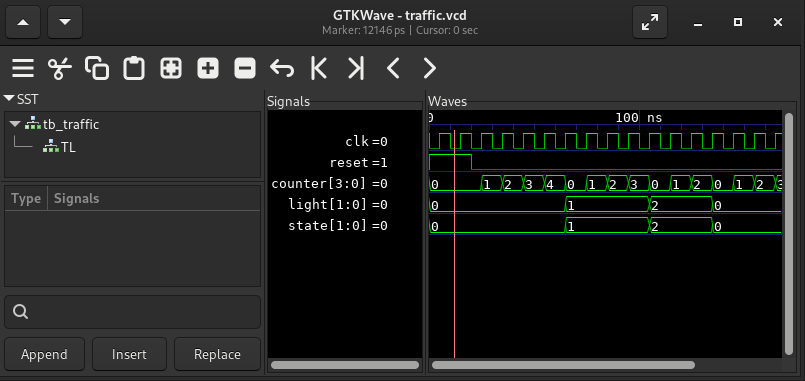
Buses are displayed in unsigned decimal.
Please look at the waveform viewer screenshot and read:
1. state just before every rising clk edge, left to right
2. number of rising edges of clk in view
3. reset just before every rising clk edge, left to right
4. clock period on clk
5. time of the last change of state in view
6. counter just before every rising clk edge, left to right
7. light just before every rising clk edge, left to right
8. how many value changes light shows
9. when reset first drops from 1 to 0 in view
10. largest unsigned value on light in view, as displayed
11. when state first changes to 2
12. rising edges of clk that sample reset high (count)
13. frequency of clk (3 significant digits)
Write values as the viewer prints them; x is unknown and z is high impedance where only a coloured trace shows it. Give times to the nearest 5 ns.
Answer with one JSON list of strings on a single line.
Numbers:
["0, 0, 0, 0, 0, 0, 0, 1, 1, 1, 1, 2, 2, 2, 0, 0, 0", "17", "1 1 0 0 0 0 0 0 0 0 0 0 0 0 0 0 0", "10 ns", "135 ns", "0, 0, 0, 1, 2, 3, 4, 0, 1, 2, 3, 0, 1, 2, 0, 1, 2", "0, 0, 0, 0, 0, 0, 0, 1, 1, 1, 1, 2, 2, 2, 0, 0, 0", "3", "20 ns", "2", "105 ns", "2", "100 MHz"]
